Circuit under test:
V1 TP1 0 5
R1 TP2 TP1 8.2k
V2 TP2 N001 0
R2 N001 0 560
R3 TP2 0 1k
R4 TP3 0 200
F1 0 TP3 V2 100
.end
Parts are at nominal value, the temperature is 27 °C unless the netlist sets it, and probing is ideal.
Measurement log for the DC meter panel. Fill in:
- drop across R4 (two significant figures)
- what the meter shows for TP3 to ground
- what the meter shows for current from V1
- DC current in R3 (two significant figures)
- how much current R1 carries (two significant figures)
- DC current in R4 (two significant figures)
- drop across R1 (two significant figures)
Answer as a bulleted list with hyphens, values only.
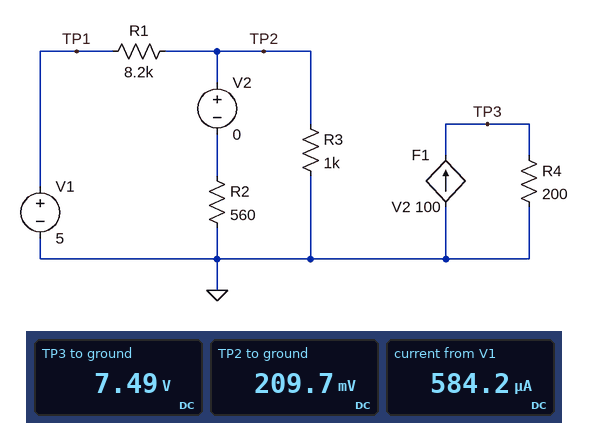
- 7.5 V
- 7.49 V
- 584.2 µA
- 210 µA
- 580 µA
- 37 mA
- 4.8 V
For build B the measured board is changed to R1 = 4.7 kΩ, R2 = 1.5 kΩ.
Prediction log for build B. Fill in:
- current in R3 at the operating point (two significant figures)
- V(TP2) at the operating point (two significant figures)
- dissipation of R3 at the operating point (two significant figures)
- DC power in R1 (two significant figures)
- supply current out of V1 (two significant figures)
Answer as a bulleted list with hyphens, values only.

- 570 µA
- 570 mV
- 320 µW
- 4.2 mW
- 940 µA
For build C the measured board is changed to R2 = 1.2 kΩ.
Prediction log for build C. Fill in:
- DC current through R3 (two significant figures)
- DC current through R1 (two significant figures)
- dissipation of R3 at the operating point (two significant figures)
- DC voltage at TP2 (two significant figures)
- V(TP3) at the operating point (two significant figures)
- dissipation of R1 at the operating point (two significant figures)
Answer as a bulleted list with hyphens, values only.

- 310 µA
- 570 µA
- 97 µW
- 310 mV
- 5.2 V
- 2.7 mW
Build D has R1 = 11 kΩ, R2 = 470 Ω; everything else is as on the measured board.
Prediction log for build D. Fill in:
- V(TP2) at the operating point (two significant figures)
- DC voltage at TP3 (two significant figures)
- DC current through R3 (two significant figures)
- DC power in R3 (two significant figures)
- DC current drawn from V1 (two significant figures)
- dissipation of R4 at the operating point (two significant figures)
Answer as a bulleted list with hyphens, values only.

- 140 mV
- 6.0 V
- 140 µA
- 20 µW
- 440 µA
- 180 mW
